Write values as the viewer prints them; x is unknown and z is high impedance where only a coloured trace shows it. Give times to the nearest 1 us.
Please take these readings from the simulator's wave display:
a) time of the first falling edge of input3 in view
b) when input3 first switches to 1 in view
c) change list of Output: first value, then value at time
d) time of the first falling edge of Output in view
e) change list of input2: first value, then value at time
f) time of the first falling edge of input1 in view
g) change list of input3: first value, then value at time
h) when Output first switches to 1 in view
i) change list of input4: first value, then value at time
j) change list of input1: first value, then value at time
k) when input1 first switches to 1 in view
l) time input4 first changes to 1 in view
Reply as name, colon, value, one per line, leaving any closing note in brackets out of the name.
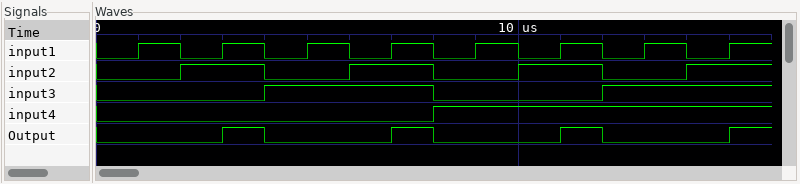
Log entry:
time of the first falling edge of input3 in view: 8 us
when input3 first switches to 1 in view: 4 us
change list of Output: first value, then value at time: 0, 1 at 3 us, 0 at 4 us, 1 at 7 us, 0 at 8 us, 1 at 11 us, 0 at 12 us, 1 at 15 us
time of the first falling edge of Output in view: 4 us
change list of input2: first value, then value at time: 0, 1 at 2 us, 0 at 4 us, 1 at 6 us, 0 at 8 us, 1 at 10 us, 0 at 12 us, 1 at 14 us
time of the first falling edge of input1 in view: 2 us
change list of input3: first value, then value at time: 0, 1 at 4 us, 0 at 8 us, 1 at 12 us
when Output first switches to 1 in view: 3 us
change list of input4: first value, then value at time: 0, 1 at 8 us
change list of input1: first value, then value at time: 0, 1 at 1 us, 0 at 2 us, 1 at 3 us, 0 at 4 us, 1 at 5 us, 0 at 6 us, 1 at 7 us, 0 at 8 us, 1 at 9 us, 0 at 10 us, 1 at 11 us, 0 at 12 us, 1 at 13 us, 0 at 14 us, 1 at 15 us
when input1 first switches to 1 in view: 1 us
time input4 first changes to 1 in view: 8 us
